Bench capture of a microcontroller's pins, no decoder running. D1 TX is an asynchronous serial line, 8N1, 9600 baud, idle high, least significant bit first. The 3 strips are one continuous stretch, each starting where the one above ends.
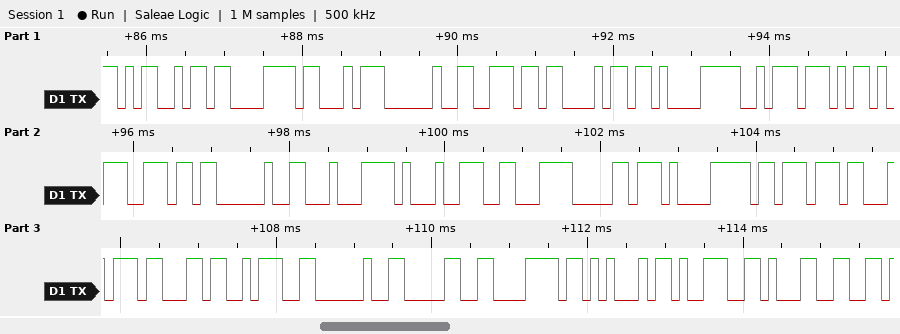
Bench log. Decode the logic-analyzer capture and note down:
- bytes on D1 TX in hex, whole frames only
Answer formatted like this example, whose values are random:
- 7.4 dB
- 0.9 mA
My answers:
- 0x4D 0xC3 0xA3 0x20 0x6E 0x68 0xE1 0xBA 0xAD 0x6E 0x20 0xC4 0x91 0xC6 0xB0 0xE1 0xBB 0xA3 0x63 0x3A 0x20 0x30 0x78 0x45 0x39 0x31
